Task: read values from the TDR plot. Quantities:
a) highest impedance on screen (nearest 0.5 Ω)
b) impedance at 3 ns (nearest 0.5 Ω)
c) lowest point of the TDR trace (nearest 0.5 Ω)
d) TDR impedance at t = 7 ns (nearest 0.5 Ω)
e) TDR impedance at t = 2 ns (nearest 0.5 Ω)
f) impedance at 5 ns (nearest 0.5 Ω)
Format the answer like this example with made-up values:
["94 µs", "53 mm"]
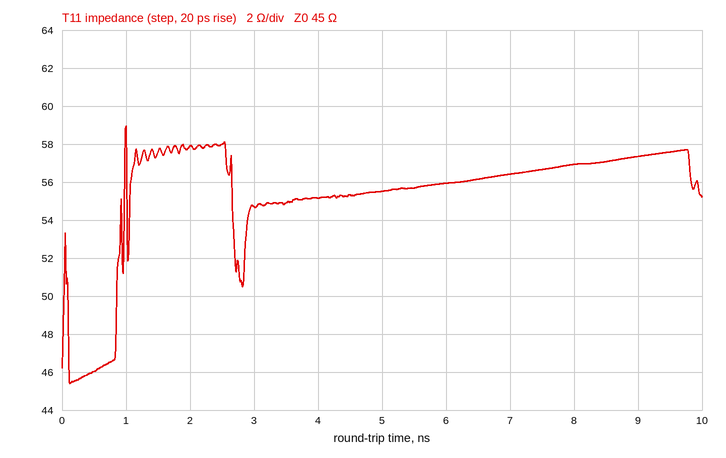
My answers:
["59.0 Ω", "54.5 Ω", "45.5 Ω", "56.5 Ω", "58.0 Ω", "55.5 Ω"]
